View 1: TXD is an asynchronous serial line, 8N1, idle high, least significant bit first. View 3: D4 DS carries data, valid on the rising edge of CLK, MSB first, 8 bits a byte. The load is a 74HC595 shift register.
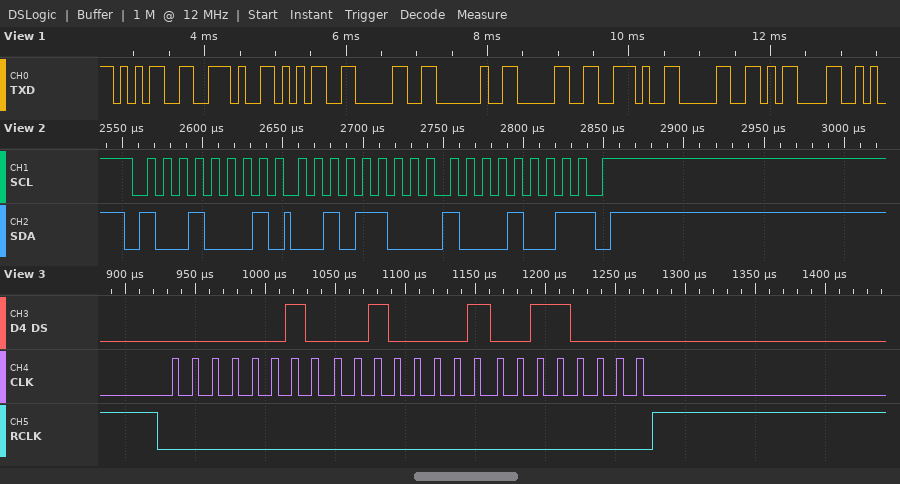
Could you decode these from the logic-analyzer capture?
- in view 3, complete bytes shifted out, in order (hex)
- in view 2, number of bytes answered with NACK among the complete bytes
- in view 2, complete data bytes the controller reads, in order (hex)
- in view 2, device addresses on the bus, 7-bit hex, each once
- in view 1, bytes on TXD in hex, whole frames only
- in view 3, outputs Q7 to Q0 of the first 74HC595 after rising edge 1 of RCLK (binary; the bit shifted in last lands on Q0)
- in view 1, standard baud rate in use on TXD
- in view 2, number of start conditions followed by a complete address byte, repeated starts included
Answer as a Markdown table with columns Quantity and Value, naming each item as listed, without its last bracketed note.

| Quantity | Value |
|---|---|
| in view 3, complete bytes shifted out, in order | 0x02 0x21 0x30 |
| in view 2, number of bytes answered with NACK among the complete bytes | 1 |
| in view 2, complete data bytes the controller reads, in order | 2C 89 |
| in view 2, device addresses on the bus, 7-bit hex, each once | 0x48 |
| in view 1, bytes on TXD in hex, whole frames only | 35 2E 35 30 20 30 2E 30 0D |
| in view 3, outputs Q7 to Q0 of the first 74HC595 after rising edge 1 of RCLK | 00110000 |
| in view 1, standard baud rate in use on TXD | 9600 baud |
| in view 2, number of start conditions followed by a complete address byte, repeated starts included | 1 |
